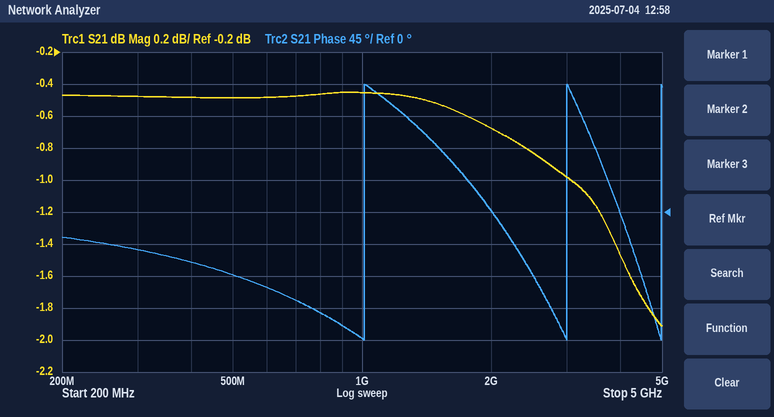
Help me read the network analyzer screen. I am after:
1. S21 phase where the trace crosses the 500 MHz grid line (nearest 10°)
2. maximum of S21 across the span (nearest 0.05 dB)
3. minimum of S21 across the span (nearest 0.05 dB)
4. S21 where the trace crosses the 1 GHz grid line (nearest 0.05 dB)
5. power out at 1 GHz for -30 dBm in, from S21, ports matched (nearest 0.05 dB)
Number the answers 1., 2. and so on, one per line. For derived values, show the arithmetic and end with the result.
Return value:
1. -90°
2. -0.45 dB
3. -1.90 dB
4. -0.45 dB
5. -30 dBm + (-0.45 dB) = -30.45 dBm
